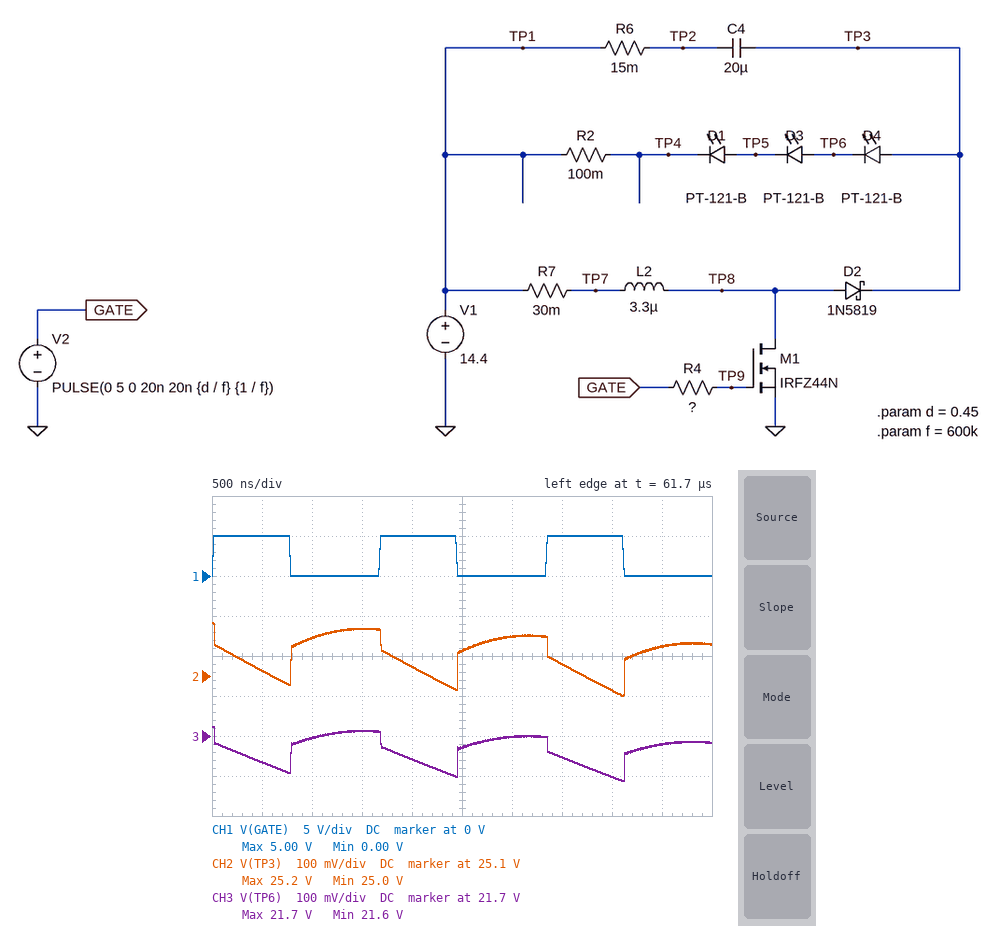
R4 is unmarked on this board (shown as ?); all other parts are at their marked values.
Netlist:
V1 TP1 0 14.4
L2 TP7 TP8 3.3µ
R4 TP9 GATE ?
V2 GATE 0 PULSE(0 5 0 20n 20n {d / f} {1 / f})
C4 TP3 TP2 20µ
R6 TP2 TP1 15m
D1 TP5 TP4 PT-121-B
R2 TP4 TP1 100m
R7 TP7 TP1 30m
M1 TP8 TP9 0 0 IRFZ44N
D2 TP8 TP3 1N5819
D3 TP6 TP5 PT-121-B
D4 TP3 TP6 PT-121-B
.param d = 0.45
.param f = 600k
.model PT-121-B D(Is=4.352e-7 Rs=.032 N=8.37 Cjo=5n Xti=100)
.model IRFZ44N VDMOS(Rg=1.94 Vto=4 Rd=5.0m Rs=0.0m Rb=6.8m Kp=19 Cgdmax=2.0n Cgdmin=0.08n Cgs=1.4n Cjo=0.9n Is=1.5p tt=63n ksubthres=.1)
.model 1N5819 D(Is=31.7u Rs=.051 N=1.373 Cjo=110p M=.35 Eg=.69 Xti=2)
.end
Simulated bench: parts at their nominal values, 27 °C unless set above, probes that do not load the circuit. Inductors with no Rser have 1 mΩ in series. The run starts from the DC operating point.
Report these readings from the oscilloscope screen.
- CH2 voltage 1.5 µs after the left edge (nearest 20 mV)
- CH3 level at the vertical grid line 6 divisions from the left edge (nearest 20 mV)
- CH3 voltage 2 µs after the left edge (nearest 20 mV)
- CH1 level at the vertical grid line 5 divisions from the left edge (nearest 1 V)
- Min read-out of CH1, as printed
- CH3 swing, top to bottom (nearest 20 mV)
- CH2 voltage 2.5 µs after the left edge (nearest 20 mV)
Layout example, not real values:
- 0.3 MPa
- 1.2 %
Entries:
- 25.22 V
- 21.70 V
- 21.64 V
- 0 V
- 0.00 V
- 140 mV
- 25.16 V
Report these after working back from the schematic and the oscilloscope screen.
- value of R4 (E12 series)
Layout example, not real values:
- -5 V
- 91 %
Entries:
- 0.68 Ω
